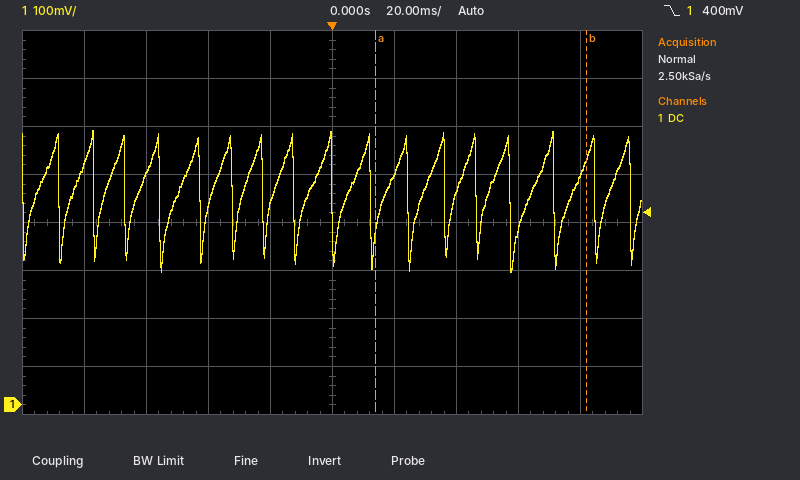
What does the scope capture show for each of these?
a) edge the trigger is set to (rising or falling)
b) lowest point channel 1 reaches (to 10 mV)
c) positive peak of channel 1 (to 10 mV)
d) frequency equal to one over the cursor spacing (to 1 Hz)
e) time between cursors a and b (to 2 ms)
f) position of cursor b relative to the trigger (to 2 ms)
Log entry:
falling
280 mV
570 mV
15 Hz
68 ms
+82 ms
